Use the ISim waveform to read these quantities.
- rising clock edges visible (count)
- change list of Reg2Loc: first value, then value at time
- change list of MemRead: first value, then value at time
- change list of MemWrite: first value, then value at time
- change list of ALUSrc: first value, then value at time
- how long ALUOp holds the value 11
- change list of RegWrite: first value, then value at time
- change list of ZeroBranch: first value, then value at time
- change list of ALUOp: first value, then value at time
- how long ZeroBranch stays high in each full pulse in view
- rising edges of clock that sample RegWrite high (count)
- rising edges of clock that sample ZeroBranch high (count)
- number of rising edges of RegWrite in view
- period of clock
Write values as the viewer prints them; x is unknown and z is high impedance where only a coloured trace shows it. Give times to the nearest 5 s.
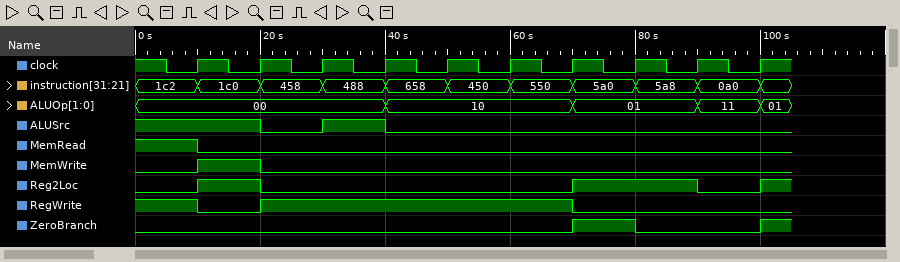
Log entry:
10
0, 1 at 10 s, 0 at 20 s, 1 at 70 s, 0 at 90 s, 1 at 100 s
1, 0 at 10 s
0, 1 at 10 s, 0 at 20 s
1, 0 at 20 s, 1 at 30 s, 0 at 40 s
10 s
1, 0 at 10 s, 1 at 20 s, 0 at 70 s
0, 1 at 70 s, 0 at 80 s, 1 at 100 s
00, 10 at 40 s, 01 at 70 s, 11 at 90 s, 01 at 100 s
10 s
6
1
1
10 s
